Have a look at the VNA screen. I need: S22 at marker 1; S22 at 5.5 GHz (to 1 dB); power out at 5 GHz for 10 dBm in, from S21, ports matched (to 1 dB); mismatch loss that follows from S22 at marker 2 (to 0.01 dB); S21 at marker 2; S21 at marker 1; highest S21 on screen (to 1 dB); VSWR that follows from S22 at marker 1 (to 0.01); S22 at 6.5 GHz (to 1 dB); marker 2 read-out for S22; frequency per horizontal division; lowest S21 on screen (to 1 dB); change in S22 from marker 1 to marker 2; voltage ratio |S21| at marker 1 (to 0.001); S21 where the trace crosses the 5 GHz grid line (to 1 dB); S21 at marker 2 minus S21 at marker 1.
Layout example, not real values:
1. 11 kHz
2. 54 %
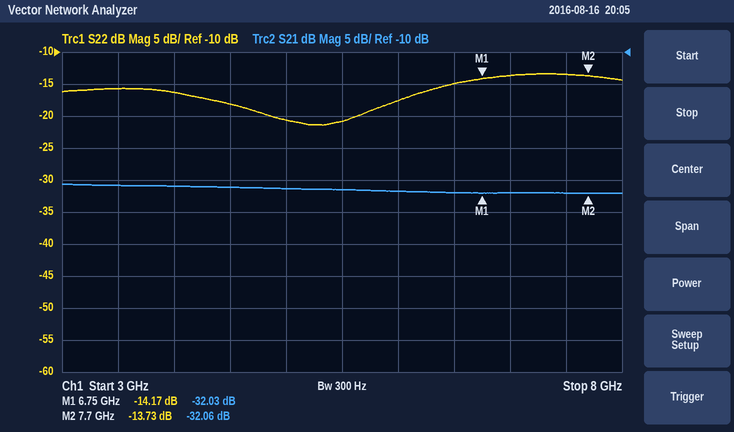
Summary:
1. -14.17 dB
2. -21 dB
3. -21 dBm
4. 0.19 dB
5. -32.06 dB
6. -32.03 dB
7. -31 dB
8. 1.49
9. -15 dB
10. -13.73 dB
11. 500 MHz
12. -32 dB
13. 0.44 dB
14. 0.025
15. -31 dB
16. -0.03 dB
